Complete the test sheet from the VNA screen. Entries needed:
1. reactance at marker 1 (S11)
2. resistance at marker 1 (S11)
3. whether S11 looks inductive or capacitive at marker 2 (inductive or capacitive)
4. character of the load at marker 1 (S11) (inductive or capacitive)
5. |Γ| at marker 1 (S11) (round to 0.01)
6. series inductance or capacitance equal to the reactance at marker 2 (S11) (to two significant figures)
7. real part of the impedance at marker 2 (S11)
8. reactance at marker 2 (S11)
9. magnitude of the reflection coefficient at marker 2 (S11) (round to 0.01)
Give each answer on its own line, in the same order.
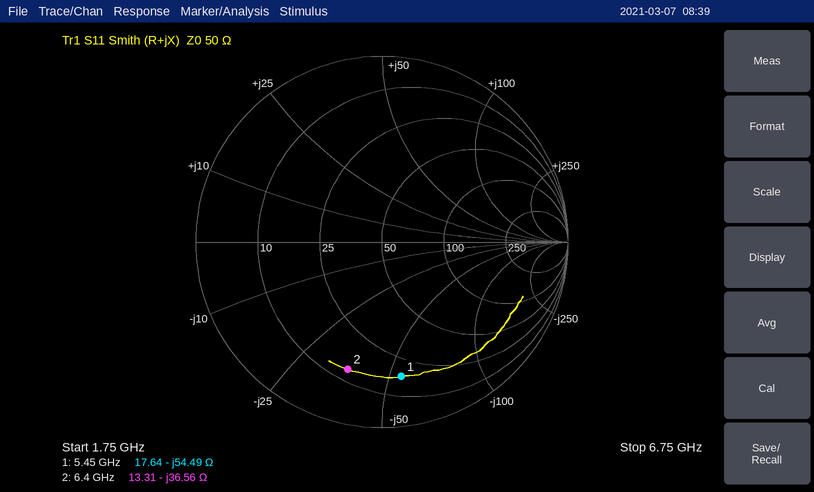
-54.49 Ω
17.64 Ω
capacitive
capacitive
0.73
680 fF
13.31 Ω
-36.56 Ω
0.71
